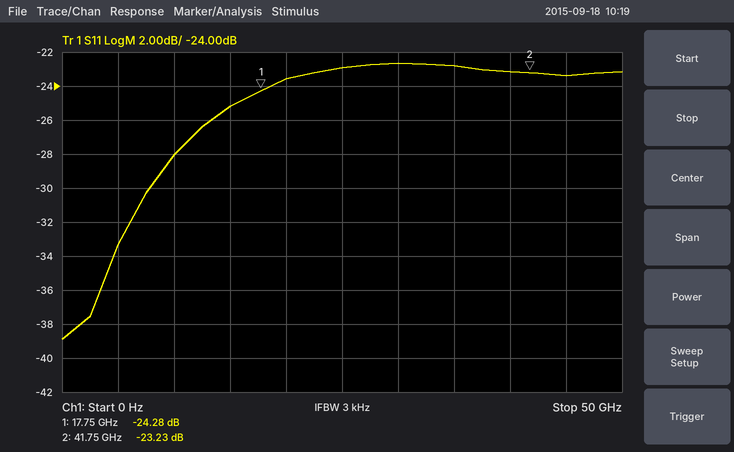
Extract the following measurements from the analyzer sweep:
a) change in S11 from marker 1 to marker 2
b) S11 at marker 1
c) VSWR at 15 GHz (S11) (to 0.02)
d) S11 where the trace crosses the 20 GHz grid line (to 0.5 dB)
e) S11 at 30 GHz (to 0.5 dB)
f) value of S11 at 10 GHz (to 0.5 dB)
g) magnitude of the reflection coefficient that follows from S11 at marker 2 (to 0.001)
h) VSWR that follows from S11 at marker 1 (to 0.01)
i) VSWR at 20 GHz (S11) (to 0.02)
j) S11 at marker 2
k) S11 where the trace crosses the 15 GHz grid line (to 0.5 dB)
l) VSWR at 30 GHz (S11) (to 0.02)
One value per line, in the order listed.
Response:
1.05 dB
-24.28 dB
1.12
-23.5 dB
-22.5 dB
-28.0 dB
0.069
1.13
1.14
-23.23 dB
-25.0 dB
1.16
